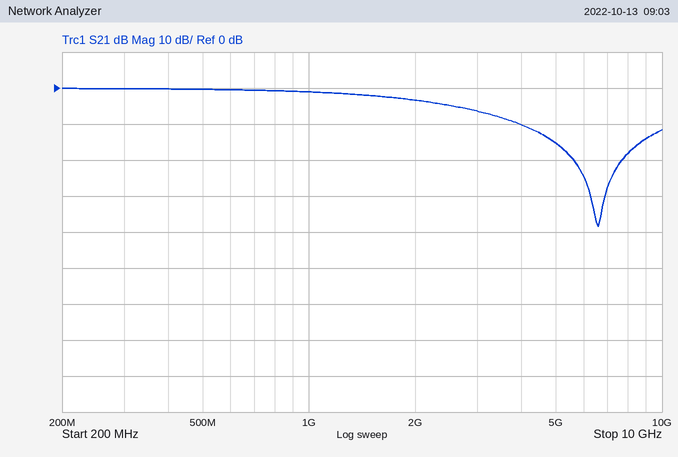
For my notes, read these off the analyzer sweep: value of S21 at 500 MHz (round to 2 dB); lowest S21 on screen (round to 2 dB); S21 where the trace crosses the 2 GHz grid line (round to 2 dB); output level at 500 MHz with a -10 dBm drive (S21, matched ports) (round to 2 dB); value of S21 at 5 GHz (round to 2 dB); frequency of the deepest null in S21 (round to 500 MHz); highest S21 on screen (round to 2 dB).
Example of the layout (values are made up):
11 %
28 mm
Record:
0 dB
-38 dB
-4 dB
-10 dBm
-16 dB
6.5 GHz
0 dB
